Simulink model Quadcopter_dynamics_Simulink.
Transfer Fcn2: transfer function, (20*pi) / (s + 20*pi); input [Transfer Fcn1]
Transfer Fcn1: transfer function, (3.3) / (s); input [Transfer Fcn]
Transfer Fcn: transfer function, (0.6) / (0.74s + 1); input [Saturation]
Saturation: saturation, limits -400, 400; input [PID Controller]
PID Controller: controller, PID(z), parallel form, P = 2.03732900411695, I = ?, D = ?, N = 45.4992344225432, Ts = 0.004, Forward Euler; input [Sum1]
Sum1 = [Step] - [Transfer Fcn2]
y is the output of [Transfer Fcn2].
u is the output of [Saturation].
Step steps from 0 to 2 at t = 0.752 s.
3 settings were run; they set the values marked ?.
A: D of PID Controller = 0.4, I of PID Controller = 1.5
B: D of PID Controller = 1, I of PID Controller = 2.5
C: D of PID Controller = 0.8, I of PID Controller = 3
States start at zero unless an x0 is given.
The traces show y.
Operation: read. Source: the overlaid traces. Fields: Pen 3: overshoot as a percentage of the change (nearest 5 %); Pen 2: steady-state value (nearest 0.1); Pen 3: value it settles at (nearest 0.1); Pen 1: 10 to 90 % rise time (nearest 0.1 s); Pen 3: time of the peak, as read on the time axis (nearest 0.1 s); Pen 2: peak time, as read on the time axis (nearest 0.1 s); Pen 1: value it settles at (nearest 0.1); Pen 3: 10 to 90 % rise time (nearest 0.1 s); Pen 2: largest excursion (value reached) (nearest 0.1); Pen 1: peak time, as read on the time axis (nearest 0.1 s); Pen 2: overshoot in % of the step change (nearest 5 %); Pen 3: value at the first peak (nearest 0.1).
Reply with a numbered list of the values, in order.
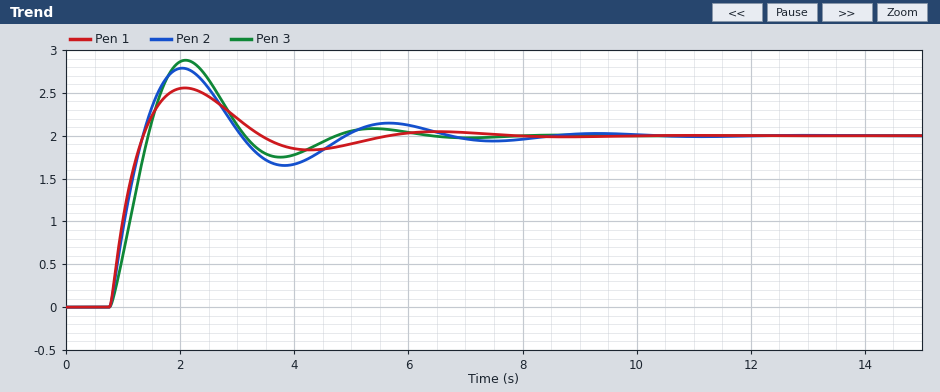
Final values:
1. 45 %
2. 2.0
3. 2.0
4. 0.4 s
5. 2.1 s
6. 2.0 s
7. 2.0
8. 0.5 s
9. 2.8
10. 2.1 s
11. 40 %
12. 2.9
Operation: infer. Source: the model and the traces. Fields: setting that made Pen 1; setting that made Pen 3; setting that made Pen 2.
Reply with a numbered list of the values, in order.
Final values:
1. B
2. A
3. C
